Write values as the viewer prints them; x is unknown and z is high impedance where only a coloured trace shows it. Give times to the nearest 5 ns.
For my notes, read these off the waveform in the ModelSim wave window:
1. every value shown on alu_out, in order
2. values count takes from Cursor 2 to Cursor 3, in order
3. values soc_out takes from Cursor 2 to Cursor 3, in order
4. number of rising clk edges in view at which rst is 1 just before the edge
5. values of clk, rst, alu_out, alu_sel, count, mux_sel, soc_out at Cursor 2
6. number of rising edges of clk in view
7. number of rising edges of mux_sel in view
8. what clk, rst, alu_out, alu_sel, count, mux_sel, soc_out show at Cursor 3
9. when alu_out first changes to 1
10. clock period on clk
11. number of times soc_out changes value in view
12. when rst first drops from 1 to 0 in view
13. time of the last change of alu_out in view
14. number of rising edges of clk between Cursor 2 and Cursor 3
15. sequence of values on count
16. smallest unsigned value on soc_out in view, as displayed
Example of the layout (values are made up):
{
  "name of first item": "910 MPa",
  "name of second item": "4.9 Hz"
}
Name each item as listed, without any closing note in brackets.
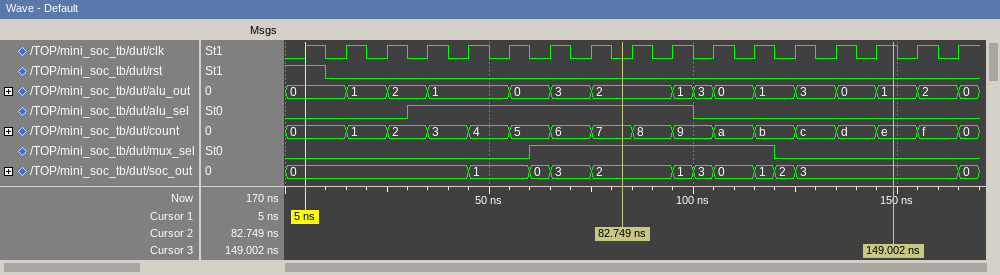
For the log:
{
  "every value shown on alu_out, in order": "0, 1, 2, 1, 0, 3, 2, 1, 3, 0, 1, 3, 0, 1, 2, 0",
  "values count takes from Cursor 2 to Cursor 3, in order": "7, 8, 9, a, b, c, d, e",
  "values soc_out takes from Cursor 2 to Cursor 3, in order": "2, 1, 3, 0, 1, 2, 3",
  "number of rising clk edges in view at which rst is 1 just before the edge": "1",
  "values of clk, rst, alu_out, alu_sel, count, mux_sel, soc_out at Cursor 2": "clk=0, rst=0, alu_out=2, alu_sel=1, count=7, mux_sel=1, soc_out=2",
  "number of rising edges of clk in view": "17",
  "number of rising edges of mux_sel in view": "1",
  "what clk, rst, alu_out, alu_sel, count, mux_sel, soc_out show at Cursor 3": "clk=1, rst=0, alu_out=1, alu_sel=0, count=e, mux_sel=0, soc_out=3",
  "when alu_out first changes to 1": "15 ns",
  "clock period on clk": "10 ns",
  "number of times soc_out changes value in view": "11",
  "when rst first drops from 1 to 0 in view": "10 ns",
  "time of the last change of alu_out in view": "165 ns",
  "number of rising edges of clk between Cursor 2 and Cursor 3": "7",
  "sequence of values on count": "0, 1, 2, 3, 4, 5, 6, 7, 8, 9, a, b, c, d, e, f, 0",
  "smallest unsigned value on soc_out in view, as displayed": "0"
}
